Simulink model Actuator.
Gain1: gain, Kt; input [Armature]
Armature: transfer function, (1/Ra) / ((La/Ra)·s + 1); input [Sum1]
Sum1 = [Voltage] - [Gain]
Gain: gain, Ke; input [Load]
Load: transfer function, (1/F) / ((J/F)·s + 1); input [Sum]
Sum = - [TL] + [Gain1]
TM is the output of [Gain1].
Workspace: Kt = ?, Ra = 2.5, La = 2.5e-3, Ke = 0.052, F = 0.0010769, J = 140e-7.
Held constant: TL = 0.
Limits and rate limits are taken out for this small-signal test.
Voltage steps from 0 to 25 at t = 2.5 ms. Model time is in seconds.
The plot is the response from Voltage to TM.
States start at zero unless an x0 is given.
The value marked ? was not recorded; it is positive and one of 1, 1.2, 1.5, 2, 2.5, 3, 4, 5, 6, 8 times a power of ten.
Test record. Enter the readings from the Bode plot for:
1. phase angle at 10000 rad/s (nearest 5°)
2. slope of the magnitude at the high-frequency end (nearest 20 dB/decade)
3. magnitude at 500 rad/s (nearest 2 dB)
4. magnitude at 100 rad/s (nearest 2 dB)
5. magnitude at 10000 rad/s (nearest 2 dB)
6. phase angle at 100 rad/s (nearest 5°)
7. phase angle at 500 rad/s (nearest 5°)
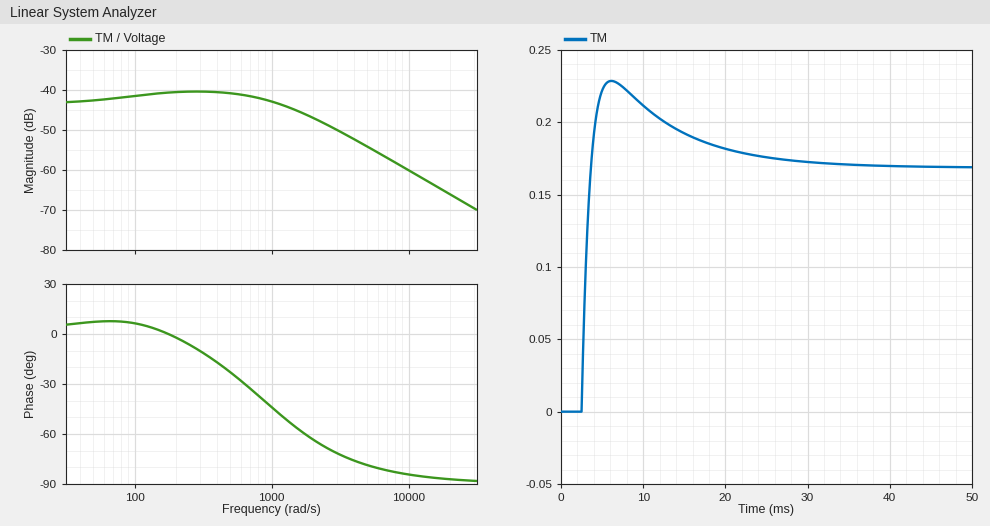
-85°
-20 dB/decade
-40 dB
-42 dB
-60 dB
5°
-25°
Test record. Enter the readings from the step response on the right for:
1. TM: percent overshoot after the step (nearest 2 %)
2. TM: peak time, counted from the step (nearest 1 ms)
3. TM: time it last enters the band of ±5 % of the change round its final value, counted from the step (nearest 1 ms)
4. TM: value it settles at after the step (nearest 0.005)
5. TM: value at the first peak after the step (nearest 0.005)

36 %
4 ms
21 ms
0.170
0.230
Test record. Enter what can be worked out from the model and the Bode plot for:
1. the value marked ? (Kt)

0.025
